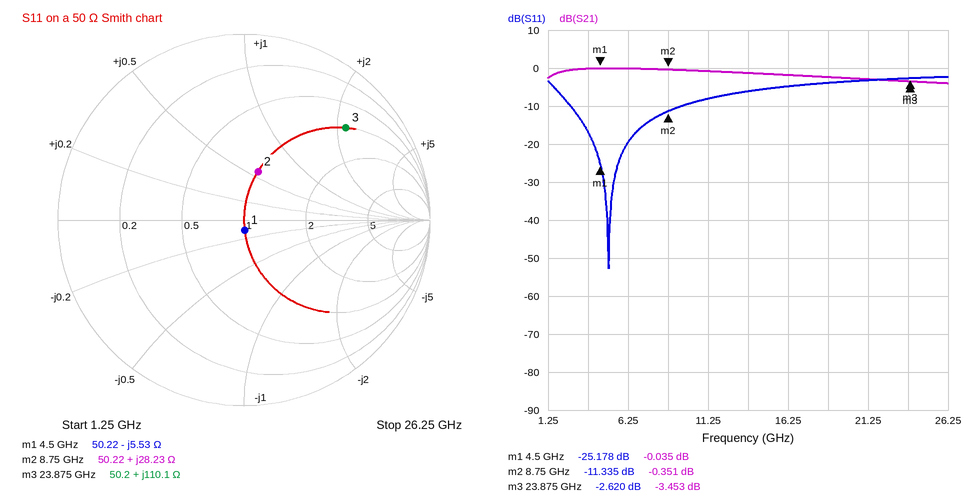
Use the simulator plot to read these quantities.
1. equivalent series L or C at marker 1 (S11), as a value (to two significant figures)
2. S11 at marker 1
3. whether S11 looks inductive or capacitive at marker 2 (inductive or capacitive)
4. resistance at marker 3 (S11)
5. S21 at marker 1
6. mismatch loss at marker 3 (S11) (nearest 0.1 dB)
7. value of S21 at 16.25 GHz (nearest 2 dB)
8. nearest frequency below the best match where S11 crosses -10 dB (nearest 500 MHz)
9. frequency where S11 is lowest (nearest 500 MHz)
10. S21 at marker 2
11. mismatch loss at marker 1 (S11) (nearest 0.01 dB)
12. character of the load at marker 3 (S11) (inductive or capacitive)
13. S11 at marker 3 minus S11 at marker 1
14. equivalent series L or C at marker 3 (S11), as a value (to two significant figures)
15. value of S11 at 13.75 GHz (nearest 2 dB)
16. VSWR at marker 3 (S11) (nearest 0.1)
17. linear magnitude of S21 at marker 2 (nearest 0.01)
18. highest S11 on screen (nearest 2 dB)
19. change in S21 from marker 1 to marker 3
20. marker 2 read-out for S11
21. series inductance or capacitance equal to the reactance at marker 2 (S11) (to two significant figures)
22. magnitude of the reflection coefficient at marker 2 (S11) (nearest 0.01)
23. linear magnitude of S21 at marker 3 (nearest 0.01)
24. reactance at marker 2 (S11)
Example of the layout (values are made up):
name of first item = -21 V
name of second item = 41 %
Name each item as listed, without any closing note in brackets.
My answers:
equivalent series L or C at marker 1 (S11), as a value = 6.4 pF
S11 at marker 1 = -25.178 dB
whether S11 looks inductive or capacitive at marker 2 = inductive
resistance at marker 3 = 50.2 Ω
S21 at marker 1 = -0.035 dB
mismatch loss at marker 3 (S11) = 3.4 dB
value of S21 at 16.25 GHz = -2 dB
nearest frequency below the best match where S11 crosses -10 dB = 2.5 GHz
frequency where S11 is lowest = 5.0 GHz
S21 at marker 2 = -0.351 dB
mismatch loss at marker 1 (S11) = 0.01 dB
character of the load at marker 3 (S11) = inductive
S11 at marker 3 minus S11 at marker 1 = 22.558 dB
equivalent series L or C at marker 3 (S11), as a value = 730 pH
value of S11 at 13.75 GHz = -6 dB
VSWR at marker 3 (S11) = 6.7
linear magnitude of S21 at marker 2 = 0.96
highest S11 on screen = -2 dB
change in S21 from marker 1 to marker 3 = -3.418 dB
marker 2 read-out for S11 = -11.335 dB
series inductance or capacitance equal to the reactance at marker 2 (S11) = 510 pH
magnitude of the reflection coefficient at marker 2 (S11) = 0.27
linear magnitude of S21 at marker 3 = 0.67
reactance at marker 2 = +28.23 Ω
